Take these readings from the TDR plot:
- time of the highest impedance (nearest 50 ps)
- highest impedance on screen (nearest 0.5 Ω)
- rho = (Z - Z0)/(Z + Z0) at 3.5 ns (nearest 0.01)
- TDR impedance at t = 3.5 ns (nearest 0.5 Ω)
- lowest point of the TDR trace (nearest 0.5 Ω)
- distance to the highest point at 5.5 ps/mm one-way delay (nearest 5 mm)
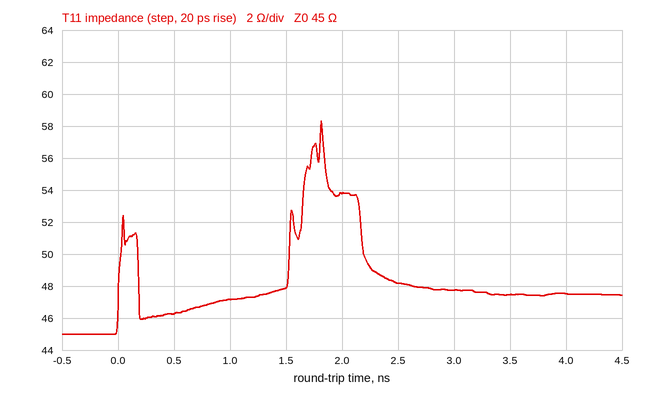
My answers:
1.80 ns
58.5 Ω
+0.03
47.5 Ω
45.0 Ω
165 mm
